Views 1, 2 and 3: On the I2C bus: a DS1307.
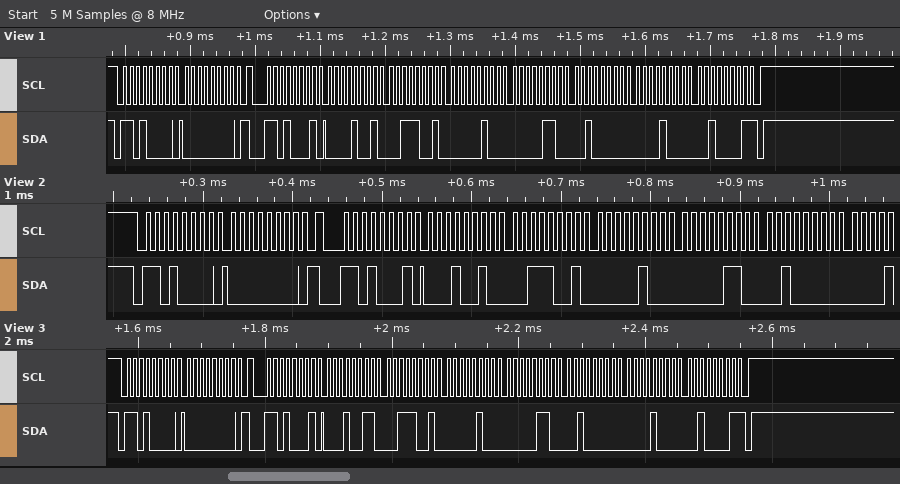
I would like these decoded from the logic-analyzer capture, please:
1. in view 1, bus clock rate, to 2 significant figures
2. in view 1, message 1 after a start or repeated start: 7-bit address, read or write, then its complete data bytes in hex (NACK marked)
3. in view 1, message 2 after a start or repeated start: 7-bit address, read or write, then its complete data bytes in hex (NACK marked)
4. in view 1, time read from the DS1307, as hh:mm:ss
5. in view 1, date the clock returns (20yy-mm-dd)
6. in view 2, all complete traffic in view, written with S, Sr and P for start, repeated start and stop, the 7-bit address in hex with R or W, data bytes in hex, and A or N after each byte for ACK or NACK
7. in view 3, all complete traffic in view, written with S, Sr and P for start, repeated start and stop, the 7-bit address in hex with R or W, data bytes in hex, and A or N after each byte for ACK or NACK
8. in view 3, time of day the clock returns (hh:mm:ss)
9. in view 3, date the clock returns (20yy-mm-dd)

100 kHz
0x68 write: 00
0x68 read: 09 39 04 06 20 08 21 NACK
04:39:09
2021-08-20
S 68W A 00 A Sr 68R A 12 A 39 A 04 A 06 A 20 A
S 68W A 00 A Sr 68R A 13 A 39 A 04 A 06 A 20 A 08 A 21 N P
04:39:13
2021-08-20
